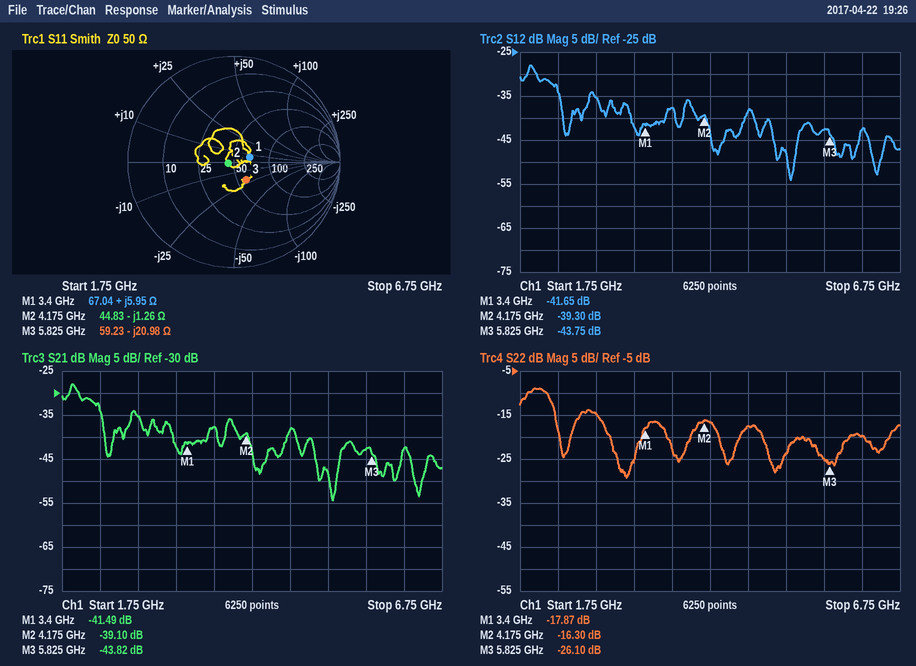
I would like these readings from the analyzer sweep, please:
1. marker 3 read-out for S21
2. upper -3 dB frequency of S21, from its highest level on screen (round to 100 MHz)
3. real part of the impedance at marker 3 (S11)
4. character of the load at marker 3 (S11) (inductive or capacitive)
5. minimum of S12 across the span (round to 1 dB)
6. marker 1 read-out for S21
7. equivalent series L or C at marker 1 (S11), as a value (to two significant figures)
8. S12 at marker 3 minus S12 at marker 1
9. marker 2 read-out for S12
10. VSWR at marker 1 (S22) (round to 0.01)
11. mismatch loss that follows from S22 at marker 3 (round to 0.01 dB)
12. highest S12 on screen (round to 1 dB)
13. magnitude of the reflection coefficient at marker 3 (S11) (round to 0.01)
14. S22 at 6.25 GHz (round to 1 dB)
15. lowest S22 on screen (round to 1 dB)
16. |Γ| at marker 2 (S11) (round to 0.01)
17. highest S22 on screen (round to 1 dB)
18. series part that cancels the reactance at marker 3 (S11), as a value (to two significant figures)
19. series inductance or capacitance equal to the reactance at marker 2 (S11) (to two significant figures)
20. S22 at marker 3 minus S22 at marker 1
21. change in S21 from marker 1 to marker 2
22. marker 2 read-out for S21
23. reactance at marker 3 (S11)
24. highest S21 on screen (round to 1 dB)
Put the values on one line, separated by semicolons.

-43.82 dB; 2.0 GHz; 59.23 Ω; capacitive; -54 dB; -41.49 dB; 280 pH; -2.10 dB; -39.30 dB; 1.29; 0.01 dB; -28 dB; 0.21; -20 dB; -29 dB; 0.06; -9 dB; 570 pH; 30 pF; -8.23 dB; 2.39 dB; -39.10 dB; -20.98 Ω; -28 dB
